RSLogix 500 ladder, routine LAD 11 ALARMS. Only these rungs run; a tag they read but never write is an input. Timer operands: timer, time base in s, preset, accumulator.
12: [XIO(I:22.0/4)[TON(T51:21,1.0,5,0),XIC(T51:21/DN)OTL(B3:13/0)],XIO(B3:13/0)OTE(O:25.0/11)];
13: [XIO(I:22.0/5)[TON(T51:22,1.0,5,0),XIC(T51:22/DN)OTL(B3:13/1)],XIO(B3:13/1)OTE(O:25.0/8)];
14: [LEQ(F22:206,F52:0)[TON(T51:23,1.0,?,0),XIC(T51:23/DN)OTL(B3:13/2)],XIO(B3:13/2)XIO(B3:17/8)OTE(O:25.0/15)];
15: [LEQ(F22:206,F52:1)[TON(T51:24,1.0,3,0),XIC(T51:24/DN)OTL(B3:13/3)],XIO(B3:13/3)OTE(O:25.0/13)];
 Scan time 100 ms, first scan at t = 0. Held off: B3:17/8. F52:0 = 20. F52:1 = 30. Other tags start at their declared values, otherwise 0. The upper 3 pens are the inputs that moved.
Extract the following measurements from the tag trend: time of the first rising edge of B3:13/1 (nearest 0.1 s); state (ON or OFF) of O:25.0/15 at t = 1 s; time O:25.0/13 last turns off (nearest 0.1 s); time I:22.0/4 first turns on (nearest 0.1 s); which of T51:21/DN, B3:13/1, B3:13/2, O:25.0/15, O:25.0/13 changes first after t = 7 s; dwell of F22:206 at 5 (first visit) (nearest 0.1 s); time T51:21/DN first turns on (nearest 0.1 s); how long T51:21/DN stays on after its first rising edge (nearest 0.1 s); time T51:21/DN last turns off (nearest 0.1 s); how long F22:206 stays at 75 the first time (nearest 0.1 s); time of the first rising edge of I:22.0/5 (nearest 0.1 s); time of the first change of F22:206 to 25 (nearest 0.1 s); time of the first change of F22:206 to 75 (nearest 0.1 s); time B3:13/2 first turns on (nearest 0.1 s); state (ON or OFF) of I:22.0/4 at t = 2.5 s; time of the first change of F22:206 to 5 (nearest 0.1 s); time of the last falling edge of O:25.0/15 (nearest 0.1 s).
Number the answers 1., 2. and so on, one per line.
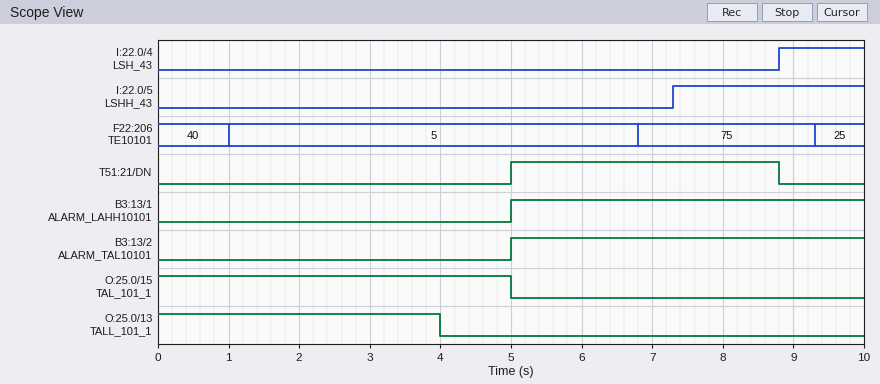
1. 5.0 s
2. ON
3. 4.0 s
4. 8.8 s
5. T51:21/DN
6. 5.8 s
7. 5.0 s
8. 3.8 s
9. 8.8 s
10. 2.5 s
11. 7.3 s
12. 9.3 s
13. 6.8 s
14. 5.0 s
15. OFF
16. 1.0 s
17. 5.0 s
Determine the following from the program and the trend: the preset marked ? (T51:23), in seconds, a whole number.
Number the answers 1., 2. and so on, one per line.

1. 4 s
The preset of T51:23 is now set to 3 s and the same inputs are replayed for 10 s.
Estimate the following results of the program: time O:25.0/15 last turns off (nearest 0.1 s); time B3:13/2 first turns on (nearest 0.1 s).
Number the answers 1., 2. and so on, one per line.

1. 4.0 s
2. 4.0 s
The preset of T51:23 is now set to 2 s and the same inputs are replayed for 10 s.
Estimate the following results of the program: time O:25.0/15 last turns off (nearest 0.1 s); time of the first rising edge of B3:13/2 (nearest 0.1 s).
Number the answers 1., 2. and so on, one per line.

1. 3.0 s
2. 3.0 s
